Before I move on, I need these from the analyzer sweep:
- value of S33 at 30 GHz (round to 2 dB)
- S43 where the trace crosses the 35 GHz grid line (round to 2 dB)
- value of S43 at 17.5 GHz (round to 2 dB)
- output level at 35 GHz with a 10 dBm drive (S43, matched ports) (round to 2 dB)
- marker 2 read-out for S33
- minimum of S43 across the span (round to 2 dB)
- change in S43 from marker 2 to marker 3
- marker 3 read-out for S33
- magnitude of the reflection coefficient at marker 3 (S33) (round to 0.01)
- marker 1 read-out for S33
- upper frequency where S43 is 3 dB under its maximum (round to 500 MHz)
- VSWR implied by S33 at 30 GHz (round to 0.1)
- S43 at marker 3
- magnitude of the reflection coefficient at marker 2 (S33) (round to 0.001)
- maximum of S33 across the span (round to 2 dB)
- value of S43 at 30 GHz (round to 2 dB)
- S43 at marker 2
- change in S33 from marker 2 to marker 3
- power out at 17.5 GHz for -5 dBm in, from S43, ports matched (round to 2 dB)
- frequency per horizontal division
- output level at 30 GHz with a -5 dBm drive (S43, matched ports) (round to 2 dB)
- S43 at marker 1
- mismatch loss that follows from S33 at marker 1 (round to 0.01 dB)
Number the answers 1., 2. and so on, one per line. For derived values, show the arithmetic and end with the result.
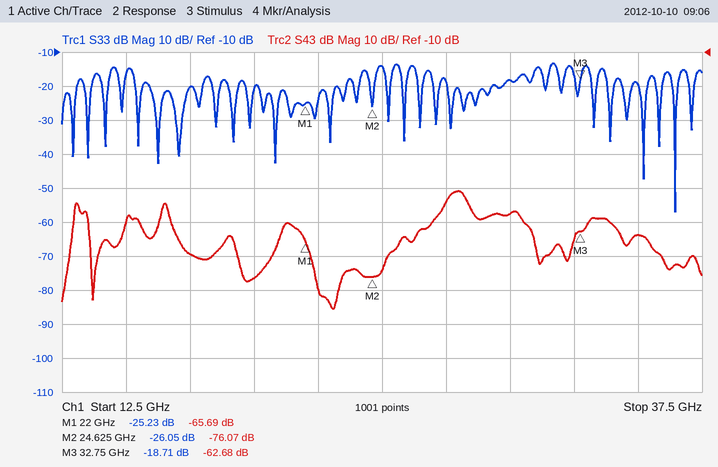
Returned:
1. -18 dB
2. -64 dB
3. -70 dB
4. 10 dBm + (-64 dB) = -54 dBm
5. -26.05 dB
6. -86 dB
7. -62.68 − (-76.07) = 13.39 dB
8. -18.71 dB
9. 10^(-18.71/20) ≈ 0.12
10. -25.23 dB
11. 28.5 GHz
12. |Γ| = 10^(-18/20) = 0.1259; VSWR = (1 + 0.1259)/(1 − 0.1259) ≈ 1.3
13. -62.68 dB
14. 10^(-26.05/20) ≈ 0.050
15. -14 dB
16. -58 dB
17. -76.07 dB
18. -18.71 − (-26.05) = 7.34 dB
19. -5 dBm + (-70 dB) = -74 dBm
20. 2.5 GHz
21. -5 dBm + (-58 dB) = -62 dBm
22. -65.69 dB
23. −10 log10(1 − 10^(-25.23/10)) ≈ 0.01 dB
